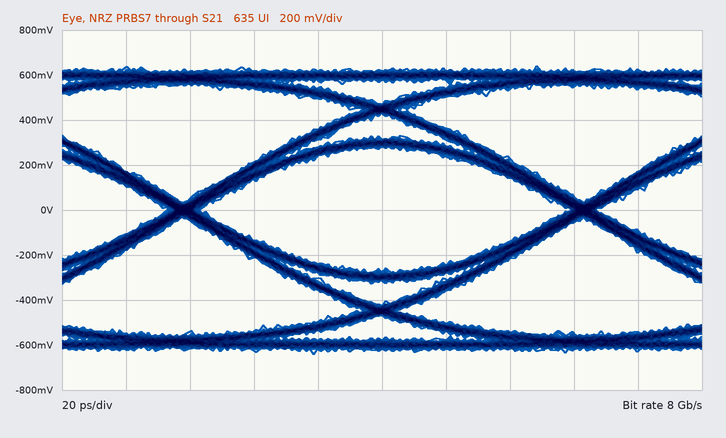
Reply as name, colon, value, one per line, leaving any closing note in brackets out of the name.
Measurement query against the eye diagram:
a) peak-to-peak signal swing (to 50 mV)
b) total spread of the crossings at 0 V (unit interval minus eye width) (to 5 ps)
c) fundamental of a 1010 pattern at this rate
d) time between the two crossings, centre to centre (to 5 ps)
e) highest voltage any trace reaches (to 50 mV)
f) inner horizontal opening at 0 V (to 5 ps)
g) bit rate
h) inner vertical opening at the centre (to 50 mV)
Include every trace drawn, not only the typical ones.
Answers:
peak-to-peak signal swing: 1.30 V
total spread of the crossings at 0 V (unit interval minus eye width): 10 ps
fundamental of a 1010 pattern at this rate: 4 GHz
time between the two crossings, centre to centre: 125 ps
highest voltage any trace reaches: 650 mV
inner horizontal opening at 0 V: 115 ps
bit rate: 8 Gb/s
inner vertical opening at the centre: 550 mV
